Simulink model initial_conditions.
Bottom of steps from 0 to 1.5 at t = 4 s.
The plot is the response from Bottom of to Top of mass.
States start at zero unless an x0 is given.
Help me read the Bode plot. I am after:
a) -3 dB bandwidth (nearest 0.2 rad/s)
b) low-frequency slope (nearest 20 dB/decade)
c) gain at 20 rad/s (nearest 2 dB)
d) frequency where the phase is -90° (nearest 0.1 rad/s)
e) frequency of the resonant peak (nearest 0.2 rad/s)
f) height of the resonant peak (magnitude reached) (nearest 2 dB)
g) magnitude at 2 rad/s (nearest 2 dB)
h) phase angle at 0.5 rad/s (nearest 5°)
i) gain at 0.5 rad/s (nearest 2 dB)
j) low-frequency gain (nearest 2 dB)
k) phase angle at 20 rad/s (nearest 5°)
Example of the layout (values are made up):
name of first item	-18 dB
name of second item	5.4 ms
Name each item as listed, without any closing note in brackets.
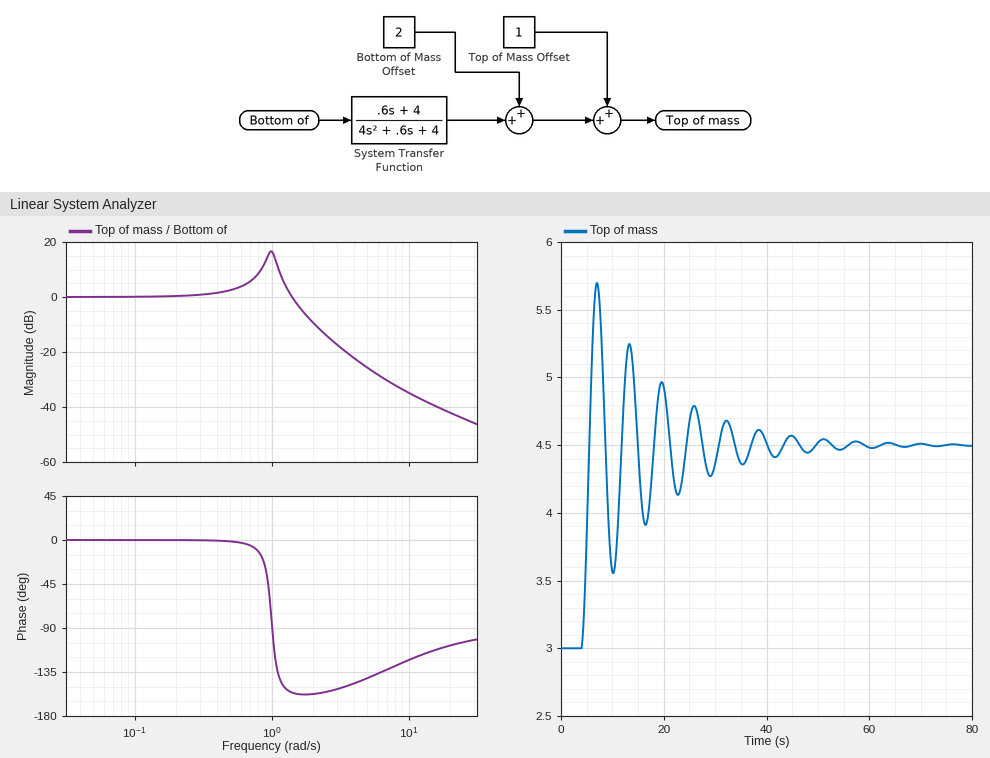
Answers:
-3 dB bandwidth	1.6 rad/s
low-frequency slope	0 dB/decade
gain at 20 rad/s	-42 dB
frequency where the phase is -90°	1.0 rad/s
frequency of the resonant peak	1.0 rad/s
height of the resonant peak (magnitude reached)	16 dB
magnitude at 2 rad/s	-10 dB
phase angle at 0.5 rad/s	0°
gain at 0.5 rad/s	2 dB
low-frequency gain	0 dB
phase angle at 20 rad/s	-110°
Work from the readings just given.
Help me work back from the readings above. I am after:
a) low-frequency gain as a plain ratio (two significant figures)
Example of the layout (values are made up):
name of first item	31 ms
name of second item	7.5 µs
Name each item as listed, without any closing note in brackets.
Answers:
low-frequency gain as a plain ratio	1.0
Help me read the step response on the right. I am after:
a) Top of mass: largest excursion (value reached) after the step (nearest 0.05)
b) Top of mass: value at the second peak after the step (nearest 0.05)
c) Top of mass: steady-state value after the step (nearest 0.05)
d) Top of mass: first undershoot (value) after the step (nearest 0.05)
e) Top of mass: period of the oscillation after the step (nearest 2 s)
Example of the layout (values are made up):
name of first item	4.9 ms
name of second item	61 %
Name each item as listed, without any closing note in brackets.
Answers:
Top of mass: largest excursion (value reached) after the step	5.70
Top of mass: value at the second peak after the step	5.25
Top of mass: steady-state value after the step	4.50
Top of mass: first undershoot (value) after the step	3.55
Top of mass: period of the oscillation after the step	6 s
